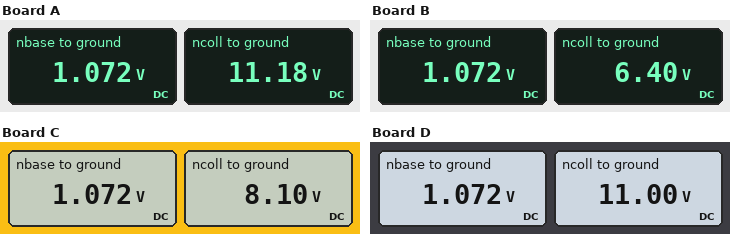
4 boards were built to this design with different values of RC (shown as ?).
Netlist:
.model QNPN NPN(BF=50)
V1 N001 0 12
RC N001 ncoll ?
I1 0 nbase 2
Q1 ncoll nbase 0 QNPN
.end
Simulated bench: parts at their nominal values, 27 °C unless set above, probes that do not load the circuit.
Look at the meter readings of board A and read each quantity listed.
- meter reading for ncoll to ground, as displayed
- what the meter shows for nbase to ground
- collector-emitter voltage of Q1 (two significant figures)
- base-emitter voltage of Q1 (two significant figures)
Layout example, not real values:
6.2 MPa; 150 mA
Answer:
11.18 V; 1.072 V; 11 V; 1.1 V
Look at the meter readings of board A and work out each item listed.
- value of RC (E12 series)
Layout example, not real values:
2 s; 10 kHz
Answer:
8.2 mΩ
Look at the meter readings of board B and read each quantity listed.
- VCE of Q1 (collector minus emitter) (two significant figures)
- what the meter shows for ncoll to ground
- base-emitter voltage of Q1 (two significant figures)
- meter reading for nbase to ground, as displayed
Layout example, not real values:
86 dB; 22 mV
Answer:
6.4 V; 6.40 V; 1.1 V; 1.072 V
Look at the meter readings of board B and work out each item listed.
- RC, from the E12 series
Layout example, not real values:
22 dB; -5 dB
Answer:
0.056 Ω
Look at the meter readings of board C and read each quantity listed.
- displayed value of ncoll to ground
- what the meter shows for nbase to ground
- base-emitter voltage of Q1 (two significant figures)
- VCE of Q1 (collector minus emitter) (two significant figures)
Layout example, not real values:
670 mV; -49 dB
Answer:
8.10 V; 1.072 V; 1.1 V; 8.1 V
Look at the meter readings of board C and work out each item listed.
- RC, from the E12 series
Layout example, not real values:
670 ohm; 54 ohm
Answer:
0.039 Ω
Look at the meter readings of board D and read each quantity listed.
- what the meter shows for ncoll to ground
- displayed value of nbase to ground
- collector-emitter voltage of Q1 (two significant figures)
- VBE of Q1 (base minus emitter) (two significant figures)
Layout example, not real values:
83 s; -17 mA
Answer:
11.00 V; 1.072 V; 11 V; 1.1 V
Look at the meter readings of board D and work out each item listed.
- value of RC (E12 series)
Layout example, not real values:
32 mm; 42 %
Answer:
0.01 Ω
